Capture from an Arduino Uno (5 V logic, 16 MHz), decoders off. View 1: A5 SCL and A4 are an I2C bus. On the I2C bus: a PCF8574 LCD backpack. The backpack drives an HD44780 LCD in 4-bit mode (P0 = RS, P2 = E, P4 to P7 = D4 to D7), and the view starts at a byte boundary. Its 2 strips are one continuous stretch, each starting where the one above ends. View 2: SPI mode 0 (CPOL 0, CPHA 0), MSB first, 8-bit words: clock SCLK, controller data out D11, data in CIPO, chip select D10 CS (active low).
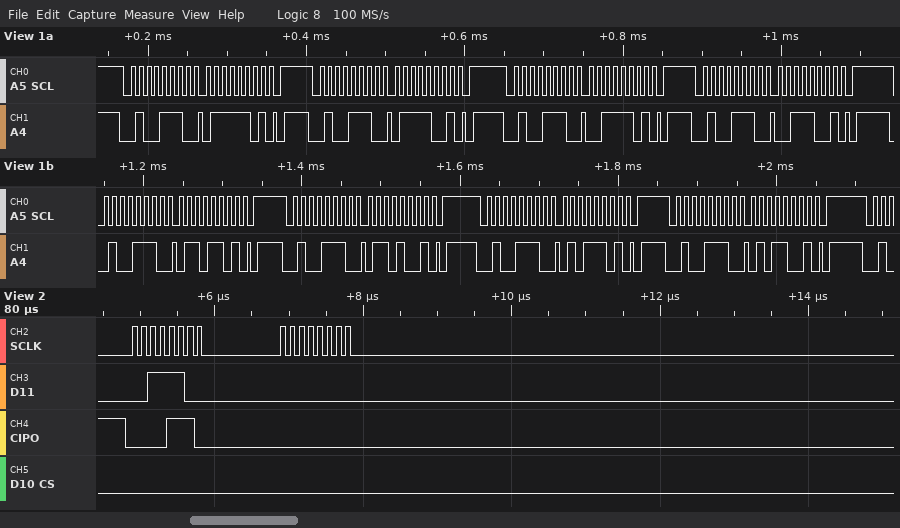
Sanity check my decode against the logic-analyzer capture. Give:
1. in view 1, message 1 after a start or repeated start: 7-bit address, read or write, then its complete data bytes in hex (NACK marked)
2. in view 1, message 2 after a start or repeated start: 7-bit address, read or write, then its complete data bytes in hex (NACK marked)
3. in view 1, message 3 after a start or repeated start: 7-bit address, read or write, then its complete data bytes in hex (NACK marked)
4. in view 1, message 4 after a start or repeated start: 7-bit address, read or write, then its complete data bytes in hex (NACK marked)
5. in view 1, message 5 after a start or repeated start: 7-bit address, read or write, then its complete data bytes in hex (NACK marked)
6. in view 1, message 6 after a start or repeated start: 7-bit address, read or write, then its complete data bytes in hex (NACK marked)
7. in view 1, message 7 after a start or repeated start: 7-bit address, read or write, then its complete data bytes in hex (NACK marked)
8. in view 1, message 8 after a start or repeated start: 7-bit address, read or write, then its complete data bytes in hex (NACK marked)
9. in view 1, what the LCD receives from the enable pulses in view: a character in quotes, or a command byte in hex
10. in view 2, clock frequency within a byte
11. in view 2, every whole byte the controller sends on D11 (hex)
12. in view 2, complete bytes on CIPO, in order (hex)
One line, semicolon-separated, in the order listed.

0x27 write: 7D; 0x27 write: 79; 0x27 write: 3D; 0x27 write: 39; 0x27 write: 6D; 0x27 write: 69; 0x27 write: 5D; 0x27 write: 59; 's' 'e'; 8 MHz; 0x3C 0x00; 0x0E 0x00
